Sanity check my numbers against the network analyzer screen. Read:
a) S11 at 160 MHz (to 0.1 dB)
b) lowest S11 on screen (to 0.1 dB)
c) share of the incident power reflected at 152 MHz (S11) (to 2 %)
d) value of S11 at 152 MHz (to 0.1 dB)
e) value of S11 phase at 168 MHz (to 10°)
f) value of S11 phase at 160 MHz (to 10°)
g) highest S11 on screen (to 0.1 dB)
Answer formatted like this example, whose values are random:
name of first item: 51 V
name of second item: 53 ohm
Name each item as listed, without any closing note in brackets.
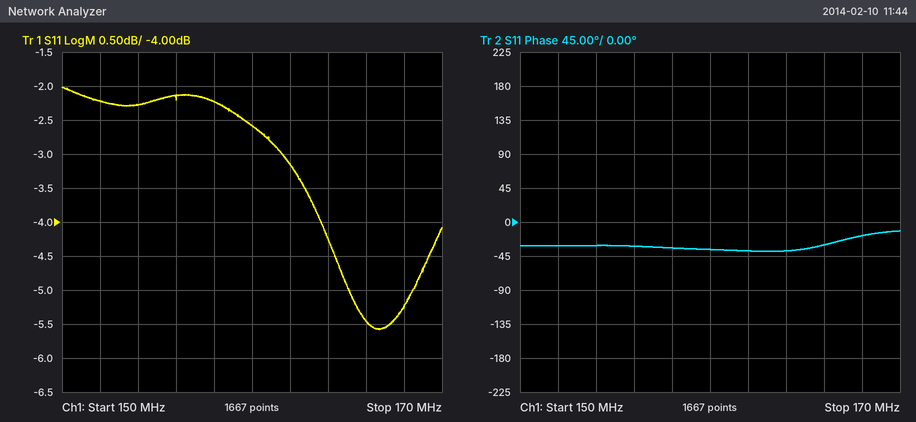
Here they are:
S11 at 160 MHz: -2.6 dB
lowest S11 on screen: -5.6 dB
share of the incident power reflected at 152 MHz (S11): 60 %
value of S11 at 152 MHz: -2.2 dB
value of S11 phase at 168 MHz: -20°
value of S11 phase at 160 MHz: -40°
highest S11 on screen: -2.0 dB
